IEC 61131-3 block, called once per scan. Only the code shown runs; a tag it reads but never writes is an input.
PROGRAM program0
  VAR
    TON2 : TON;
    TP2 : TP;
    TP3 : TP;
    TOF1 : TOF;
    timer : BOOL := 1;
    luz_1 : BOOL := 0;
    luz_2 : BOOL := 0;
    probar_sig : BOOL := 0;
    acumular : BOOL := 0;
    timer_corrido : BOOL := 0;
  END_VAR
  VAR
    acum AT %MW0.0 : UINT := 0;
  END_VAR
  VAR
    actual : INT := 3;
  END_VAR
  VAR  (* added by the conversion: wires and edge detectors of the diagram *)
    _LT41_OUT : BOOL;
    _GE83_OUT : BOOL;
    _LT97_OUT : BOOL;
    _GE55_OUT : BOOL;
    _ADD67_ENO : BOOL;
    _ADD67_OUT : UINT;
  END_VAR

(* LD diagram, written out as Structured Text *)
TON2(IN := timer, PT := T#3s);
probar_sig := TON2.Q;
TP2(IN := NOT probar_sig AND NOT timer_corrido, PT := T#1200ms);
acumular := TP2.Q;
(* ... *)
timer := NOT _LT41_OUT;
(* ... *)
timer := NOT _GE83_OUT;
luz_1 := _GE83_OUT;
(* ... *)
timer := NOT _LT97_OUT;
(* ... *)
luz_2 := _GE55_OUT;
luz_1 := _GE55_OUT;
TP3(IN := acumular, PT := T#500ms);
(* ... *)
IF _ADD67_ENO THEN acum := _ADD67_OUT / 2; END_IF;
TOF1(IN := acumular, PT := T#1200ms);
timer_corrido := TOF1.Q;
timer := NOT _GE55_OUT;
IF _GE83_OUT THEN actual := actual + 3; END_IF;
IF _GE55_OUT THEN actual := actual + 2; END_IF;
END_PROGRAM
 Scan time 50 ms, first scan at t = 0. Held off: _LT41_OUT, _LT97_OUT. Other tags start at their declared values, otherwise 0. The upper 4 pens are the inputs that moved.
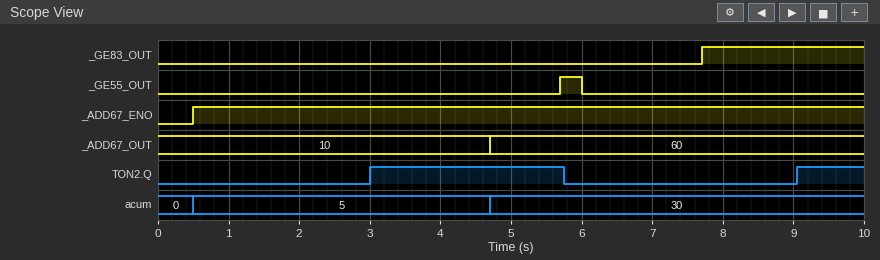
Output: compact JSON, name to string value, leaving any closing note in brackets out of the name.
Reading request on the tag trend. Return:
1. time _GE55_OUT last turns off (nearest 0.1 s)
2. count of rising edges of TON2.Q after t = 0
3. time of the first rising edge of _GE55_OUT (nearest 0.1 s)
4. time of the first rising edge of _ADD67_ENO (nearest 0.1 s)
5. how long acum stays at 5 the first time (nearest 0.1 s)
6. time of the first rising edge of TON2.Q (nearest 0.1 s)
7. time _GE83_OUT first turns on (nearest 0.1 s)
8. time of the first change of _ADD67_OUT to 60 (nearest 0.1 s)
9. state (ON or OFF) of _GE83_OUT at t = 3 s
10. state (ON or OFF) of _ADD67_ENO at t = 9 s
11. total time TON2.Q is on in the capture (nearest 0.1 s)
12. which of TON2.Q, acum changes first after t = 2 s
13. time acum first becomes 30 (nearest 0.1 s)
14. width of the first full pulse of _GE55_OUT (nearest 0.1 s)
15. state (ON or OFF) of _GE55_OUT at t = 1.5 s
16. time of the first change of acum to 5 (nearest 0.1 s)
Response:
{"time _GE55_OUT last turns off": "6.0 s", "count of rising edges of TON2.Q after t = 0": "2", "time of the first rising edge of _GE55_OUT": "5.7 s", "time of the first rising edge of _ADD67_ENO": "0.5 s", "how long acum stays at 5 the first time": "4.2 s", "time of the first rising edge of TON2.Q": "3.0 s", "time _GE83_OUT first turns on": "7.7 s", "time of the first change of _ADD67_OUT to 60": "4.7 s", "state (ON or OFF) of _GE83_OUT at t = 3 s": "OFF", "state (ON or OFF) of _ADD67_ENO at t = 9 s": "ON", "total time TON2.Q is on in the capture": "3.7 s", "which of TON2.Q, acum changes first after t = 2 s": "TON2.Q", "time acum first becomes 30": "4.7 s", "width of the first full pulse of _GE55_OUT": "0.3 s", "state (ON or OFF) of _GE55_OUT at t = 1.5 s": "OFF", "time of the first change of acum to 5": "0.5 s"}
